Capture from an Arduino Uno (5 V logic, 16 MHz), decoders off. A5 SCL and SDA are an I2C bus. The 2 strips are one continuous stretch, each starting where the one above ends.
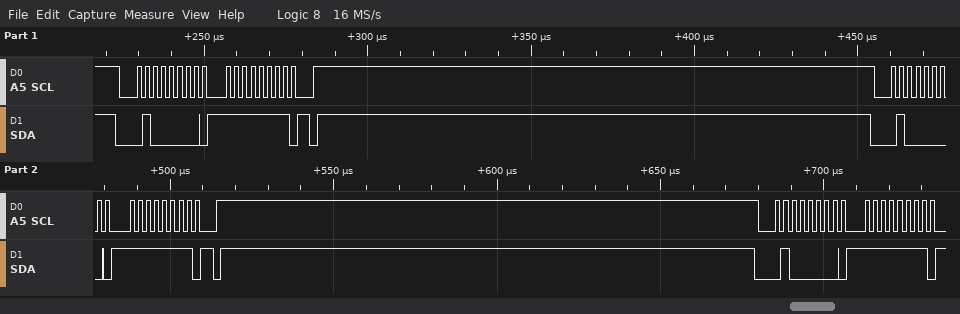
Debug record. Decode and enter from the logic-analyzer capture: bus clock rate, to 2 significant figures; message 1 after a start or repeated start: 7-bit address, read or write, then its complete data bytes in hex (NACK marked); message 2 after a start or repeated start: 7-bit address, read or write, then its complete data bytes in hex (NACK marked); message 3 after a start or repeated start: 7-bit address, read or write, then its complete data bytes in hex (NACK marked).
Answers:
400 kHz
0x20 write: FF
0x20 write: FF
0x20 write: FF
